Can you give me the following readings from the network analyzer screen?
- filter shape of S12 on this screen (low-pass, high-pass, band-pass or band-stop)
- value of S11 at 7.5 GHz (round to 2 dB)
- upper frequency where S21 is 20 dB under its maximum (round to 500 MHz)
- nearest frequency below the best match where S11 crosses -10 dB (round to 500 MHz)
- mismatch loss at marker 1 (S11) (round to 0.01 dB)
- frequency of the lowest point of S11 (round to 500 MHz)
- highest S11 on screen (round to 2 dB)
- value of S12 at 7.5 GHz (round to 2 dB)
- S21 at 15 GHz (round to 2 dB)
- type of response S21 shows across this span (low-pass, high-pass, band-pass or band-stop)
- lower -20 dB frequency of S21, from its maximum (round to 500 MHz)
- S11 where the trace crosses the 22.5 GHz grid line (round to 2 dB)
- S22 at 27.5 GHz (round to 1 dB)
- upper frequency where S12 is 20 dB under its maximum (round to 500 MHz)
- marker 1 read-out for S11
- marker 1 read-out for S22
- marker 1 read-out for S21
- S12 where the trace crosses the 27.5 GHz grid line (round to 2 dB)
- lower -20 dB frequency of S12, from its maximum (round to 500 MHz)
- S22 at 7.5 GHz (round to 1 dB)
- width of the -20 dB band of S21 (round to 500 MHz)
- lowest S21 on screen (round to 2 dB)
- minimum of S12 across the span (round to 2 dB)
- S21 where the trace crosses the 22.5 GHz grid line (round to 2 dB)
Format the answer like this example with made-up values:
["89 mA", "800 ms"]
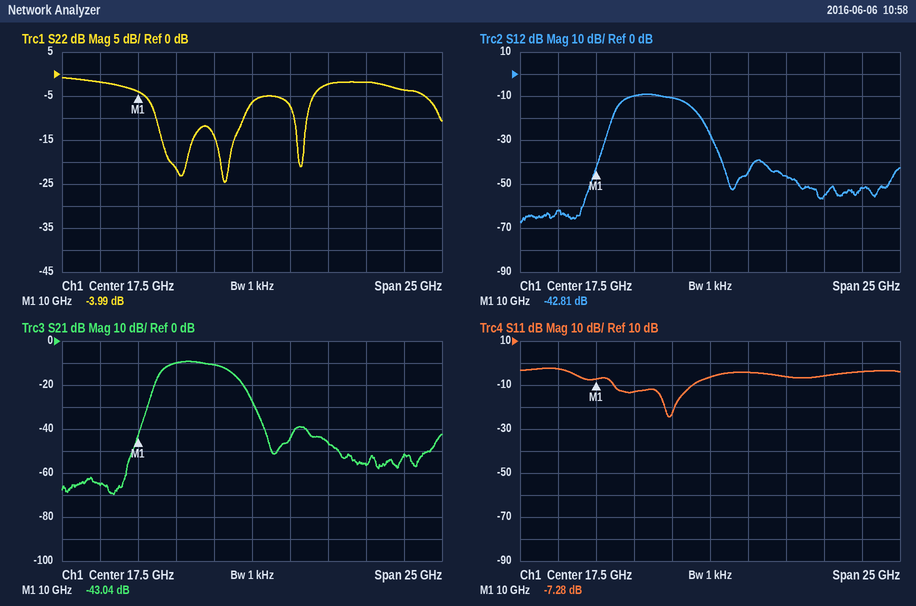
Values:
["band-pass", "-2 dB", "17.5 GHz", "11.0 GHz", "0.90 dB", "15.0 GHz", "-2 dB", "-62 dB", "-10 dB", "band-pass", "10.5 GHz", "-6 dB", "-4 dB", "17.5 GHz", "-7.28 dB", "-3.99 dB", "-43.04 dB", "-52 dB", "10.5 GHz", "-2 dB", "7.0 GHz", "-70 dB", "-68 dB", "-46 dB"]
